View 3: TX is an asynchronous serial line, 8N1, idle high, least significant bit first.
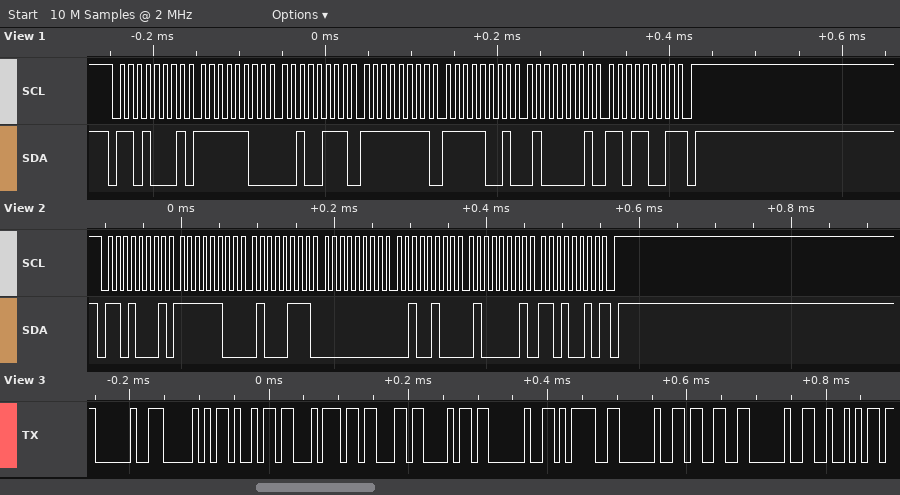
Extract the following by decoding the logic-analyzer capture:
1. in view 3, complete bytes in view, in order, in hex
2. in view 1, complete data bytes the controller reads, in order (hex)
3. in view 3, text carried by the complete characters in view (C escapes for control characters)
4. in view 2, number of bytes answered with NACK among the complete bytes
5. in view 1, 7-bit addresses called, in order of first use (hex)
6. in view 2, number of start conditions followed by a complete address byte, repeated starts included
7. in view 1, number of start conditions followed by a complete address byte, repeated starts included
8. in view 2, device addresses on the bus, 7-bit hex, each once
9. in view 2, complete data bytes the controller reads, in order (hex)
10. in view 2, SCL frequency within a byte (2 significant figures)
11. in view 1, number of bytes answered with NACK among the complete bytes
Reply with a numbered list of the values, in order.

1. 20 50 69 74 63 68 20 3D 20 33 20 52
2. FC 27 FF F9 41 D9
3. " Pitch = 3 R"
4. 1
5. 0x68
6. 1
7. 1
8. 0x68
9. FC 47 00 24 41 D2
10. 100 kHz
11. 1
